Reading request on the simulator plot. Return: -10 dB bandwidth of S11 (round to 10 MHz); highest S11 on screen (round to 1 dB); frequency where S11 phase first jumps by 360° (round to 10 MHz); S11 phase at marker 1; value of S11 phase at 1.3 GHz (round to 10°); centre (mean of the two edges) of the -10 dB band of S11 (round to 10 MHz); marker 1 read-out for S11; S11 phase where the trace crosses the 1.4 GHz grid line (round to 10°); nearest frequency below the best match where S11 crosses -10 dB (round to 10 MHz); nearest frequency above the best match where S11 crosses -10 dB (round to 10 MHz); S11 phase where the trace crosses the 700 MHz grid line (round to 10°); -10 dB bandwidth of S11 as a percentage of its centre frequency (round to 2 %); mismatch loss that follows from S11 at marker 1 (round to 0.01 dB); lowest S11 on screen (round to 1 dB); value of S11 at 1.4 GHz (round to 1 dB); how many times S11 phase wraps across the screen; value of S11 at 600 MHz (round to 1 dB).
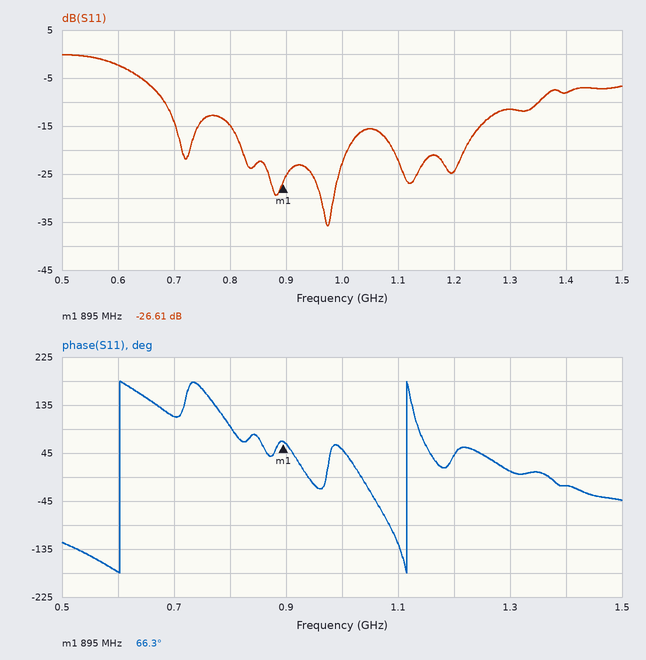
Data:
670 MHz
0 dB
600 MHz
66.3°
10°
1.02 GHz
-26.61 dB
-20°
680 MHz
1.35 GHz
110°
66 %
0.01 dB
-36 dB
-8 dB
2
-2 dB
